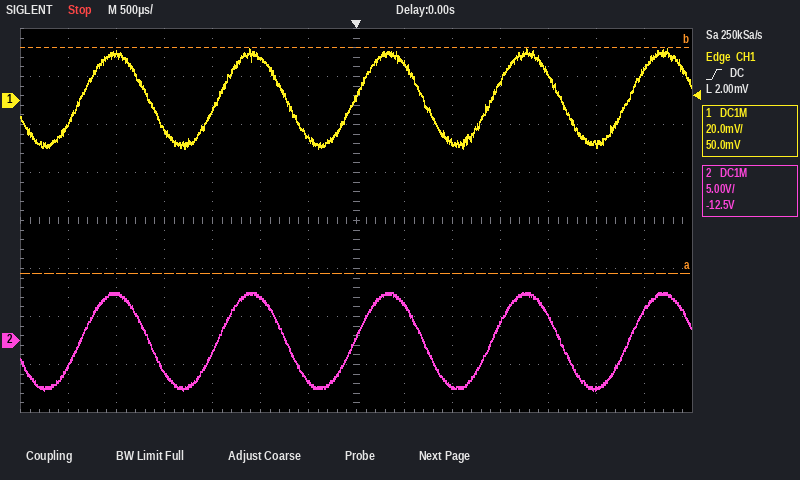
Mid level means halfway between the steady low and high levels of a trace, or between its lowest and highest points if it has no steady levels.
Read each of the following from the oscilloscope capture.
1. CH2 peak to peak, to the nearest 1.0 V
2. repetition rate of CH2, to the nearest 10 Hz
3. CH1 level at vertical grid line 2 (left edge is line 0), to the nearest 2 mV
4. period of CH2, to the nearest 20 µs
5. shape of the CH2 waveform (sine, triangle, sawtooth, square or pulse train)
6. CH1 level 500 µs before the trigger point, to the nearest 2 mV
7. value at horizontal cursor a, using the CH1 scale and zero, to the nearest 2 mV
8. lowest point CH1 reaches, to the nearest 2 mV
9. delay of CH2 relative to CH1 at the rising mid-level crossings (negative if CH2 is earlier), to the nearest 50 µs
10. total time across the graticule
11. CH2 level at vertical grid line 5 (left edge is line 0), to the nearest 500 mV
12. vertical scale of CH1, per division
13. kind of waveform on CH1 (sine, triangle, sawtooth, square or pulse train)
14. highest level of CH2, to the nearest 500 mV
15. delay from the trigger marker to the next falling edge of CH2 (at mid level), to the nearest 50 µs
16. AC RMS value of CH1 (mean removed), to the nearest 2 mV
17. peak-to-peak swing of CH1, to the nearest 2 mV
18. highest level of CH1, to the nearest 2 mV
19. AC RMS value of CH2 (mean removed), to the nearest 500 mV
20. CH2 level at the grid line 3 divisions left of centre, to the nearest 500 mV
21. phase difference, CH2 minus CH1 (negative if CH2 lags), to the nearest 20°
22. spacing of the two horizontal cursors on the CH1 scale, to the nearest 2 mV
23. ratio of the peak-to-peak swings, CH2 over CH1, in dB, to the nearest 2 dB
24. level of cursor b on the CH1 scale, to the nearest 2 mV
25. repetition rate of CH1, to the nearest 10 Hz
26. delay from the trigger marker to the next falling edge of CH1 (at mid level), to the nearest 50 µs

10.0 V
700 Hz
20 mV
1.42 ms
sine
-16 mV
-72 mV
-20 mV
0 µs
7 ms
4.5 V
20 mV
sine
5.0 V
700 µs
14 mV
42 mV
22 mV
3.5 V
-1.5 V
0°
94 mV
48 dB
22 mV
700 Hz
700 µs
